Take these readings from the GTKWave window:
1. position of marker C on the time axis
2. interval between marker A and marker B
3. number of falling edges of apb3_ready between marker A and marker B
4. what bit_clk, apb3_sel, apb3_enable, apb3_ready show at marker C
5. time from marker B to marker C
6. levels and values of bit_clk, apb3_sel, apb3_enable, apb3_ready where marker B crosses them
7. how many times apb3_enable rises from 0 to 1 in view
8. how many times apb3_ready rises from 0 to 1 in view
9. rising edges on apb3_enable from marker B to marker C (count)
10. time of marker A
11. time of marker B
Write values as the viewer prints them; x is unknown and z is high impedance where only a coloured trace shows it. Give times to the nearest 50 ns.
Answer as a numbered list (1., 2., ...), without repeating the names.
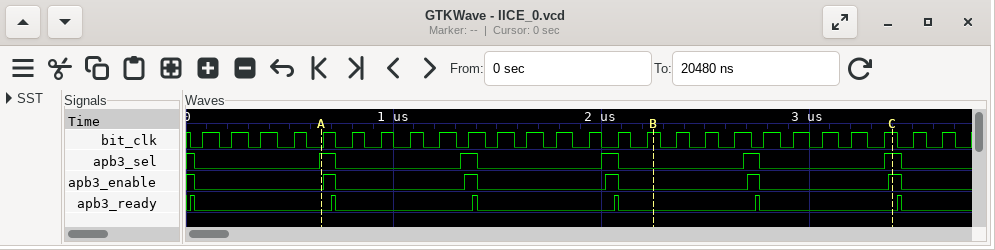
1. 3400 ns
2. 1600 ns
3. 3
4. bit_clk=1, apb3_sel=1, apb3_enable=1, apb3_ready=0
5. 1150 ns
6. bit_clk=1, apb3_sel=0, apb3_enable=0, apb3_ready=0
7. 5
8. 6
9. 2
10. 650 ns
11. 2250 ns
